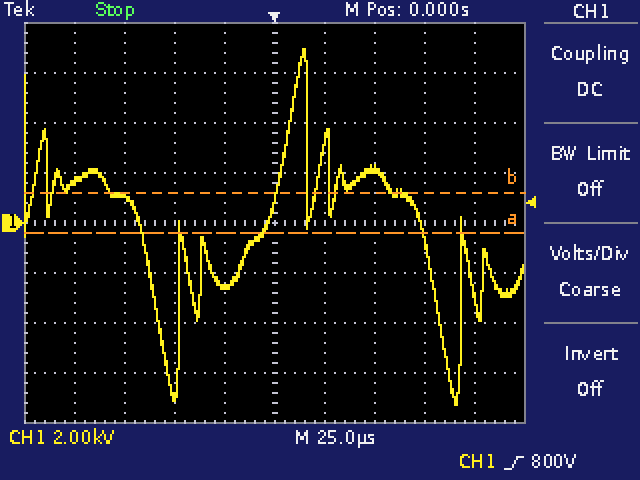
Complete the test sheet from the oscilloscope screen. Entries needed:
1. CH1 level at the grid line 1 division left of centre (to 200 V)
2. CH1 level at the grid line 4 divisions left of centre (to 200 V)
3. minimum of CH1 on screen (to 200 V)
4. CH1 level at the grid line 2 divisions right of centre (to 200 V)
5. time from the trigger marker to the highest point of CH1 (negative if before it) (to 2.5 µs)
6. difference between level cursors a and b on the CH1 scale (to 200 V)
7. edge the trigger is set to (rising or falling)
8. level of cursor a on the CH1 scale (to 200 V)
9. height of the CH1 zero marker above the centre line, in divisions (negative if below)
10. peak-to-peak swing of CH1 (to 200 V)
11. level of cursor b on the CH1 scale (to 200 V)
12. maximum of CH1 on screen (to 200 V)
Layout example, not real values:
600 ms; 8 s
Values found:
-2.6 kV; 1.6 kV; -7.2 kV; 2.2 kV; +15.0 µs; 1.6 kV; rising; -400 V; 0.0 div; 14.2 kV; 1.2 kV; 7.0 kV
